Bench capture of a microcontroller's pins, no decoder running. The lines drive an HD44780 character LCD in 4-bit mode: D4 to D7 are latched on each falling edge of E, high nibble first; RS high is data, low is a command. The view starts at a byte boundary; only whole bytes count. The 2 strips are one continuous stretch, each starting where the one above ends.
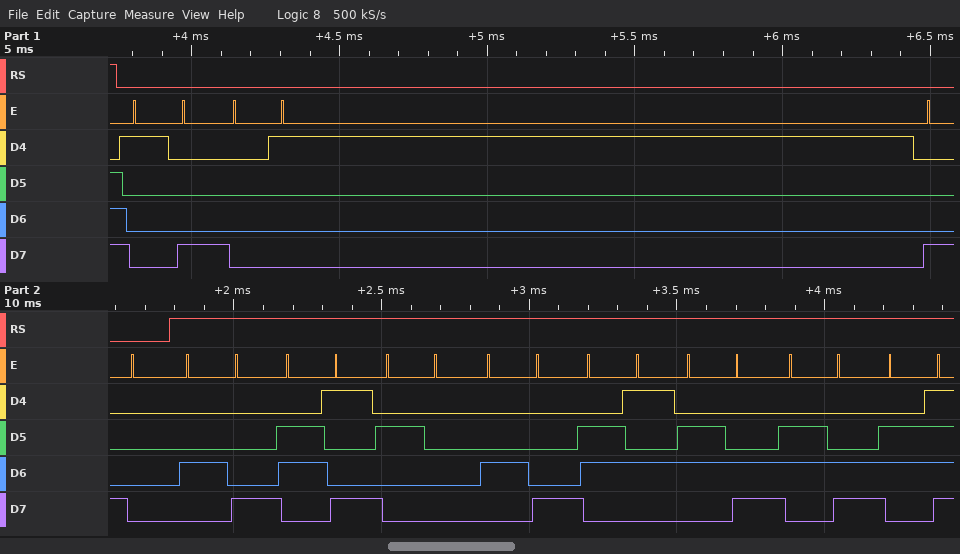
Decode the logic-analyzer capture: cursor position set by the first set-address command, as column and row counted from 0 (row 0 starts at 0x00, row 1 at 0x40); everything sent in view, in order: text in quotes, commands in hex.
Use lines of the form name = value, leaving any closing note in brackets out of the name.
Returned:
cursor position set by the first set-address command, as column and row counted from 0 = column 0, row 0
everything sent in view, in order: text in quotes, commands in hex = 0x18 0x01 0x80 "Hi Hello"
